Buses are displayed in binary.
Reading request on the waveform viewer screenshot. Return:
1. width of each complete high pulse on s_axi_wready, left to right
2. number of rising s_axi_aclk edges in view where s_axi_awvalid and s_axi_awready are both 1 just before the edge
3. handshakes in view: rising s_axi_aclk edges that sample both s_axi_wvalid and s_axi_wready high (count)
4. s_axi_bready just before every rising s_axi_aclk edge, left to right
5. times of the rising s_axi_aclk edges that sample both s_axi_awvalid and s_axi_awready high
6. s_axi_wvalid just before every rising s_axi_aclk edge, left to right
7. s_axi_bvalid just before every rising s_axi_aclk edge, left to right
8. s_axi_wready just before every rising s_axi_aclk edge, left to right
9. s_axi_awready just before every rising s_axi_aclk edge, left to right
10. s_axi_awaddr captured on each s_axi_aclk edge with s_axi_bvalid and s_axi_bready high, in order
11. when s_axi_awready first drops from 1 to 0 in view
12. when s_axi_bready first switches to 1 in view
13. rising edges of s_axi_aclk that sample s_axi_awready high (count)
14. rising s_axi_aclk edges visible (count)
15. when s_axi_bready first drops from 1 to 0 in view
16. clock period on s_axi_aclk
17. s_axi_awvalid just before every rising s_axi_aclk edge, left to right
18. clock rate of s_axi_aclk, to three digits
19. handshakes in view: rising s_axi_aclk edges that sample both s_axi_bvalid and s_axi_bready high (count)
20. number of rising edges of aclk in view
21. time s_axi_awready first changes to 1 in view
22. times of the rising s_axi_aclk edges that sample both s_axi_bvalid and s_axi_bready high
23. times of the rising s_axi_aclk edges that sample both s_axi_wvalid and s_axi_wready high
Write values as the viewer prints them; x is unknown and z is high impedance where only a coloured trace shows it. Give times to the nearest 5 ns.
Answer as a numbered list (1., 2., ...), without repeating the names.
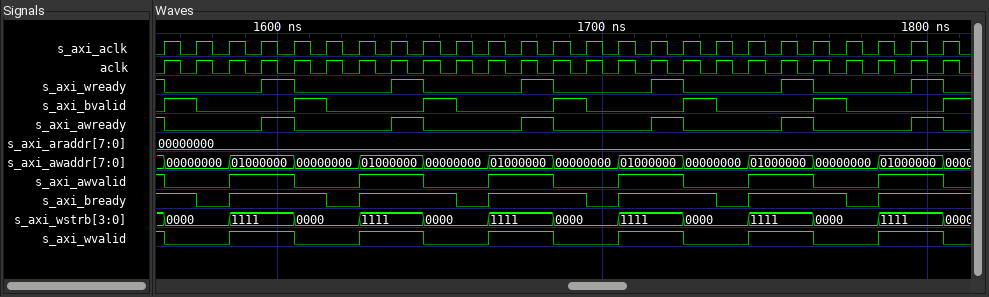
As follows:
1. 10 ns, 10 ns, 10 ns, 10 ns, 10 ns, 10 ns
2. 7
3. 7
4. 1 1 0 1 1 1 0 1 1 1 0 1 1 1 0 1 1 1 0 1 1 1 0 1 1
5. 1565 ns, 1605 ns, 1645 ns, 1685 ns, 1725 ns, 1765 ns, 1805 ns
6. 1 0 0 1 1 0 0 1 1 0 0 1 1 0 0 1 1 0 0 1 1 0 0 1 1
7. 0 1 0 0 0 1 0 0 0 1 0 0 0 1 0 0 0 1 0 0 0 1 0 0 0
8. 1 0 0 0 1 0 0 0 1 0 0 0 1 0 0 0 1 0 0 0 1 0 0 0 1
9. 1 0 0 0 1 0 0 0 1 0 0 0 1 0 0 0 1 0 0 0 1 0 0 0 1
10. 00000000, 00000000, 00000000, 00000000, 00000000, 00000000
11. 1565 ns
12. 1585 ns
13. 7
14. 25
15. 1575 ns
16. 10 ns
17. 1 0 0 1 1 0 0 1 1 0 0 1 1 0 0 1 1 0 0 1 1 0 0 1 1
18. 100 MHz
19. 6
20. 25
21. 1595 ns
22. 1575 ns, 1615 ns, 1655 ns, 1695 ns, 1735 ns, 1775 ns
23. 1565 ns, 1605 ns, 1645 ns, 1685 ns, 1725 ns, 1765 ns, 1805 ns
